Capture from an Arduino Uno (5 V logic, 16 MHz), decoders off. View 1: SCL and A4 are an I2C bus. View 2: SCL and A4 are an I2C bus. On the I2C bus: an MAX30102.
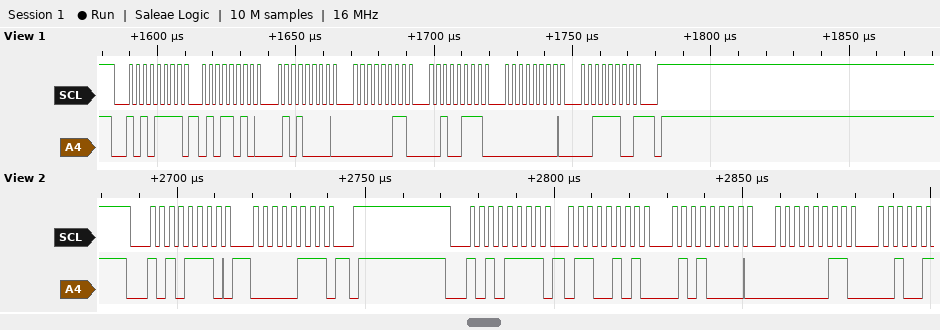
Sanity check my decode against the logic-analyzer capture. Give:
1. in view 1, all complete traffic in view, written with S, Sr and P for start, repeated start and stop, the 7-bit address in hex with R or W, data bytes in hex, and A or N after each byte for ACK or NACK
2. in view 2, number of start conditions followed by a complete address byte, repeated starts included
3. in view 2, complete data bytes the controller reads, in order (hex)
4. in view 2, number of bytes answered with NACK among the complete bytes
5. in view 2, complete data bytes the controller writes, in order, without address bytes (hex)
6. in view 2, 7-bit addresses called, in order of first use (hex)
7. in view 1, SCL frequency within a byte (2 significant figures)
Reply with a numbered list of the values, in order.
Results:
1. S 57R A 5A A 50 A 03 A 27 A 00 A 3C N P
2. 2
3. 65 50 03
4. 0
5. 07
6. 0x57
7. 400 kHz
